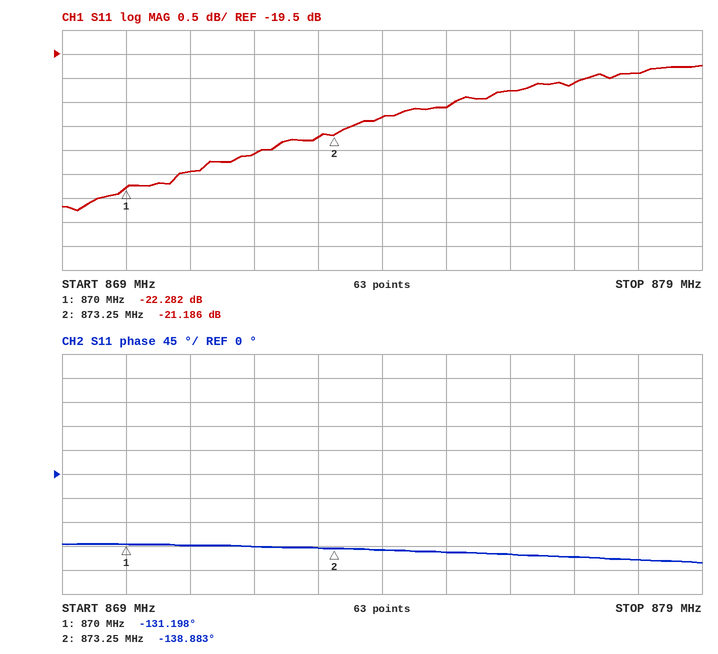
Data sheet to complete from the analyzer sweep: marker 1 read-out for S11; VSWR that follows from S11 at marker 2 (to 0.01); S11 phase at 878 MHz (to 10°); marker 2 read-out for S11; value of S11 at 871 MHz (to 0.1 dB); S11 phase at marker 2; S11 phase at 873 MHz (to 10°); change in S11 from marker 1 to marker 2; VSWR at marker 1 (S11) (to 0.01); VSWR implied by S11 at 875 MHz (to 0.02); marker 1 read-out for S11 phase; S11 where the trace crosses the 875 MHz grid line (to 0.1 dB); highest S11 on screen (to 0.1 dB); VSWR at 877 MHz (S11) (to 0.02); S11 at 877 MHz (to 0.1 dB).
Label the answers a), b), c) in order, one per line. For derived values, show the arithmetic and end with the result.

a) -22.282 dB
b) (1 + 0.0872)/(1 − 0.0872) ≈ 1.19
c) -160°
d) -21.186 dB
e) -21.9 dB
f) -138.883°
g) -140°
h) -21.186 − (-22.282) = 1.096 dB
i) (1 + 0.0769)/(1 − 0.0769) ≈ 1.17
j) |Γ| = 10^(-20.6/20) = 0.0933; VSWR = (1 + 0.0933)/(1 − 0.0933) ≈ 1.21, so 1.20 to the nearest 0.02
k) -131.198°
l) -20.6 dB
m) -19.7 dB
n) |Γ| = 10^(-20.1/20) = 0.0989; VSWR = (1 + 0.0989)/(1 − 0.0989) ≈ 1.22
o) -20.1 dB
